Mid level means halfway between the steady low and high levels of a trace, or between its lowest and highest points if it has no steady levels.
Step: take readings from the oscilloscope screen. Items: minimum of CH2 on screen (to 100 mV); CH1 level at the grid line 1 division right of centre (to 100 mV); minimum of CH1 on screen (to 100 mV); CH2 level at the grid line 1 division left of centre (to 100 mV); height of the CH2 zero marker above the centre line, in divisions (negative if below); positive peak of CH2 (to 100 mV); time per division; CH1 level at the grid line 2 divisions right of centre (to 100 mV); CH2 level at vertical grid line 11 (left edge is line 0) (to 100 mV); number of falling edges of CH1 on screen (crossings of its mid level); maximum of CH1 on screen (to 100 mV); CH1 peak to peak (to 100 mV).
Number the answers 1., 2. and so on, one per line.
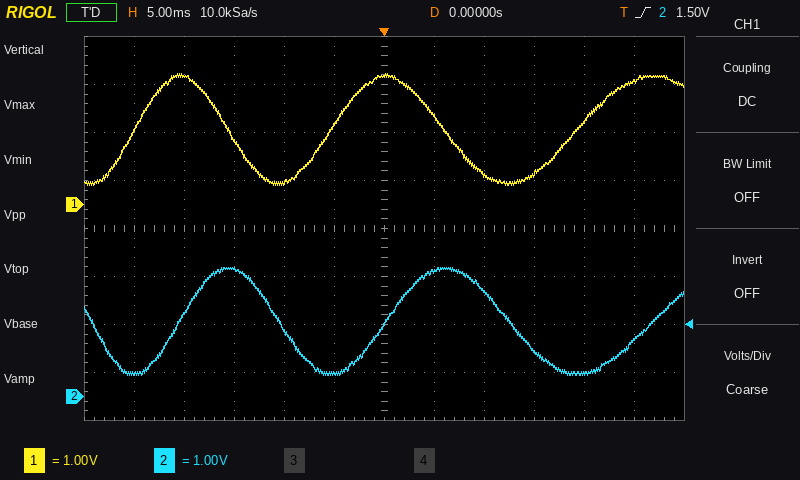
1. 400 mV
2. 1.8 V
3. 400 mV
4. 500 mV
5. -3.5 div
6. 2.7 V
7. 5 ms
8. 600 mV
9. 1.2 V
10. 2
11. 2.7 V
12. 2.3 V
